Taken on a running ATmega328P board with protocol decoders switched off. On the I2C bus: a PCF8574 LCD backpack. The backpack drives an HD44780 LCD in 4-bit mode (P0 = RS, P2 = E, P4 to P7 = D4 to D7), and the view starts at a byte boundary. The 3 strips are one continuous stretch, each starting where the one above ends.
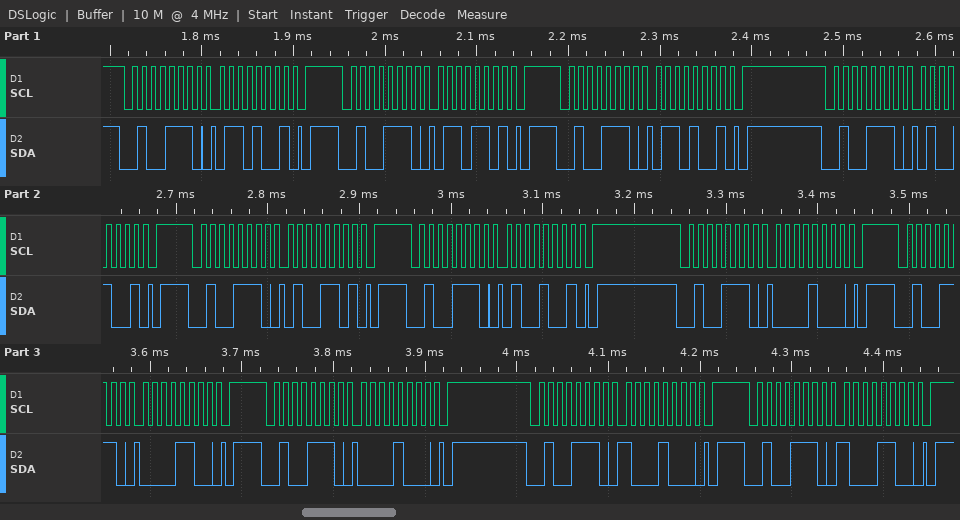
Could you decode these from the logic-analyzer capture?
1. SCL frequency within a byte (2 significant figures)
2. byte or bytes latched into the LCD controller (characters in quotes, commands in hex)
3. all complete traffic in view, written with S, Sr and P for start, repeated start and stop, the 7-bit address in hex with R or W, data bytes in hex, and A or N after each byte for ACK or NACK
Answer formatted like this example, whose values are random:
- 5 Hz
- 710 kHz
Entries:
- 100 kHz
- 'd'
- S 27W A 69 A P S 27W A 6D A P S 27W A 69 A P S 27W A 49 A P S 27W A 4D A P S 27W A 49 A P S 27W A 08 A P S 27W A 0C A P S 27W A 08 A P S 27W A 88 A P S 27W A 8C A P
